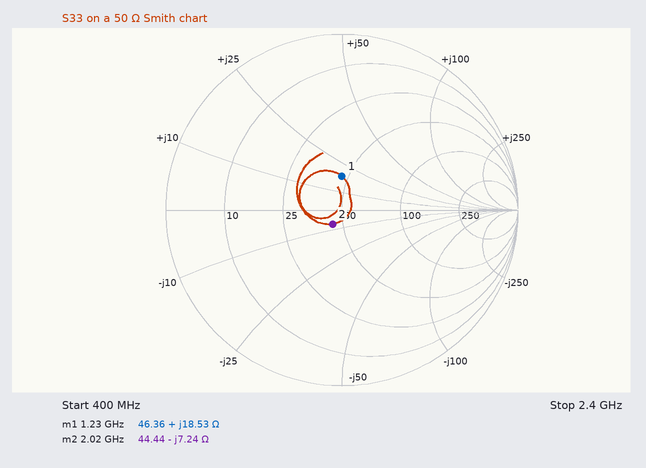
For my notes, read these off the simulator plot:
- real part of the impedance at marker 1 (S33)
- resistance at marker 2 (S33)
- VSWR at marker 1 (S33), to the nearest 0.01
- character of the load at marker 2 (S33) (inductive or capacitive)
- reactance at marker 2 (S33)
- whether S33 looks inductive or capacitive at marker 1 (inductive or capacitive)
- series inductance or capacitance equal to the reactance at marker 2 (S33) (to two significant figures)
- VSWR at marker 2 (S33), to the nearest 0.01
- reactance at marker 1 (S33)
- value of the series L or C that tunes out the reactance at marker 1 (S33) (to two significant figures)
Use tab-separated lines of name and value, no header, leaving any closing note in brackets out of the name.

real part of the impedance at marker 1	46.36 Ω
resistance at marker 2	44.44 Ω
VSWR at marker 1 (S33), to the nearest 0.01	1.48
character of the load at marker 2 (S33)	capacitive
reactance at marker 2	-7.24 Ω
whether S33 looks inductive or capacitive at marker 1	inductive
series inductance or capacitance equal to the reactance at marker 2 (S33)	11 pF
VSWR at marker 2 (S33), to the nearest 0.01	1.21
reactance at marker 1	+18.53 Ω
value of the series L or C that tunes out the reactance at marker 1 (S33)	7.0 pF
